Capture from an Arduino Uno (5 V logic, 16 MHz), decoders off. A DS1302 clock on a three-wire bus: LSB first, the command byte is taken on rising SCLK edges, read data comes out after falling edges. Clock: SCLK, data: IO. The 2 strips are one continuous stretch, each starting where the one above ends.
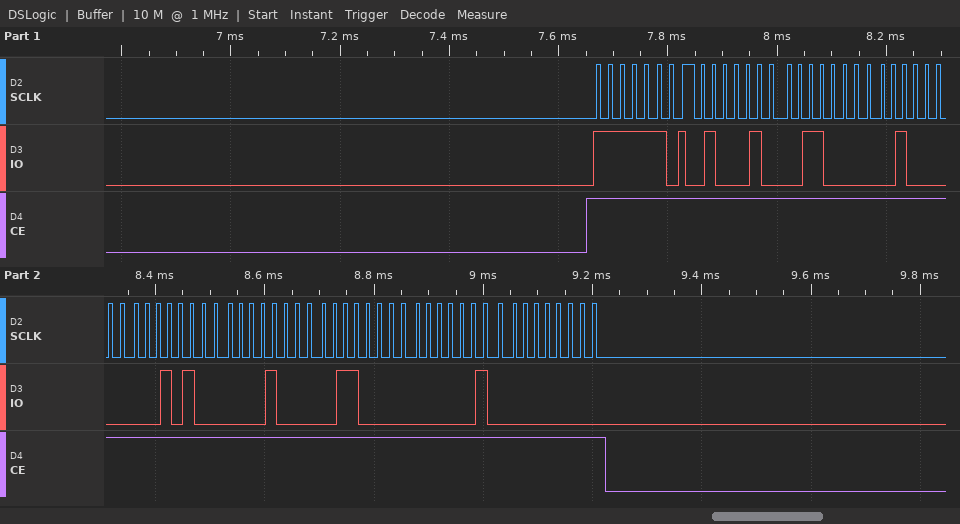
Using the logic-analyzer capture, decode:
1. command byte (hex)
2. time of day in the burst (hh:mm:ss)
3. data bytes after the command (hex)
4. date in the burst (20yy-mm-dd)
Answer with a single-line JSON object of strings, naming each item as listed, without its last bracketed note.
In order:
{"command byte": "0xBF", "time of day in the burst": "02:06:22", "data bytes after the command": "22 06 02 14 08 06 20 00", "date in the burst": "2020-08-14"}
